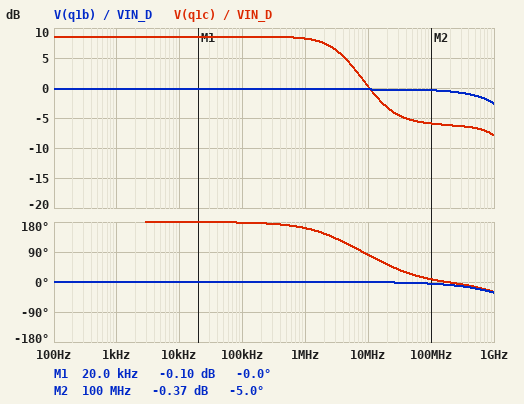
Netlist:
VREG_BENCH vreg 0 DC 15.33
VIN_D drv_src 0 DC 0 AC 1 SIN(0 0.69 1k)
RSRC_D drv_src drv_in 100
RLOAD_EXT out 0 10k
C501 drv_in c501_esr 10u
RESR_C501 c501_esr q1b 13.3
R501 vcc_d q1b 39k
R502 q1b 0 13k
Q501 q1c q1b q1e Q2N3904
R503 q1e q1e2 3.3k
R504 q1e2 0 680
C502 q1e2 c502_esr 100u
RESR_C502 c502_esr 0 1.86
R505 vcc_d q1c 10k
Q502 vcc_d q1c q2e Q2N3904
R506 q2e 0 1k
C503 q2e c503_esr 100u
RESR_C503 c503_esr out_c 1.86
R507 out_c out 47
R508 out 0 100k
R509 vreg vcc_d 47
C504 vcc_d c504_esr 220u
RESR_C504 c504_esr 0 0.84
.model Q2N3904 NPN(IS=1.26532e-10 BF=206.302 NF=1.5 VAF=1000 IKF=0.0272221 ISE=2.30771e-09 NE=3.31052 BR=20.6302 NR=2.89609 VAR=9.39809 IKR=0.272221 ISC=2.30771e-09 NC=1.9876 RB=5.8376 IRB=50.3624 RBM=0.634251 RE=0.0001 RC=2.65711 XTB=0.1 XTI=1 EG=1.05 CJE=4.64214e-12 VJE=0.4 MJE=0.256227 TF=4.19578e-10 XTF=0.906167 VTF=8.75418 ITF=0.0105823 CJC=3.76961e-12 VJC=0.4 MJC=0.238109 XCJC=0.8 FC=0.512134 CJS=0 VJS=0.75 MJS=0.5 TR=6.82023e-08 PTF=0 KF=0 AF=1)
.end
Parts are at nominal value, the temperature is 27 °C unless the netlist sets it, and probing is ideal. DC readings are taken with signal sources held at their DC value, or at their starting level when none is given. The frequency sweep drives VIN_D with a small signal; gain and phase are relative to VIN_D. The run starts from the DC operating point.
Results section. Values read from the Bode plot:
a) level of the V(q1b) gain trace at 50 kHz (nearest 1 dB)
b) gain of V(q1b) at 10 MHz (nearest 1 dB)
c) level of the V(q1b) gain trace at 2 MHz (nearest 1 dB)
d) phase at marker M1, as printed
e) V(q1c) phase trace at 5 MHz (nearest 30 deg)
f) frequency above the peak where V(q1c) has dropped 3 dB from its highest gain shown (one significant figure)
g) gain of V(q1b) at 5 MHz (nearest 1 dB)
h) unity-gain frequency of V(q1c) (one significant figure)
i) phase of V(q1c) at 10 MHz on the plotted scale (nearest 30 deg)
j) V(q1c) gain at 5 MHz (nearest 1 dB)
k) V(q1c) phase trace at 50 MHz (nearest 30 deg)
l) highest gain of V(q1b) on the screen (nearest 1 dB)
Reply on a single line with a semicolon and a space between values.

0 dB; 0 dB; 0 dB; -0.0 deg; 120 deg; 4 MHz; 0 dB; 10 MHz; 90 deg; 4 dB; 30 deg; 0 dB
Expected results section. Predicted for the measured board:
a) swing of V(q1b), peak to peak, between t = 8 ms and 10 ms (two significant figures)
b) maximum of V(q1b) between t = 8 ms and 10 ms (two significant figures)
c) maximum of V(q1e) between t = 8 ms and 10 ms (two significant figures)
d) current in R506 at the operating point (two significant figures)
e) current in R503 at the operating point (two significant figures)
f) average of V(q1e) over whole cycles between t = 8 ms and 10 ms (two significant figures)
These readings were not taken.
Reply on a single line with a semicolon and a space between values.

1.4 V; 4.4 V; 3.7 V; 6.2 mA; 770 µA; 3.1 V
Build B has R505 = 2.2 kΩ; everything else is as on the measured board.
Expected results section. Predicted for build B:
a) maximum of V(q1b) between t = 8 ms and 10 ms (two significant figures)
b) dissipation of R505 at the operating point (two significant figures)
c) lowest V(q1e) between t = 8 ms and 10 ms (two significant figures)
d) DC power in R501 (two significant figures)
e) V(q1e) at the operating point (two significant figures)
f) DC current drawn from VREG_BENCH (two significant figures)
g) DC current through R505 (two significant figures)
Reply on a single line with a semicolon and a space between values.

4.3 V; 1.6 mW; 2.3 V; 3.2 mW; 3.0 V; 13 mA; 850 µA
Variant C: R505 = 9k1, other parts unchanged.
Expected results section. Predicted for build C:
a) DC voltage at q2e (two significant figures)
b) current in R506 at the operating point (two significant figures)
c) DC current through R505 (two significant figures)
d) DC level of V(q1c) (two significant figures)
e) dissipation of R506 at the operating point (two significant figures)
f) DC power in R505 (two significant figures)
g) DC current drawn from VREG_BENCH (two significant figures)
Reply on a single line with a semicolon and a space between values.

6.8 V; 6.8 mA; 820 µA; 7.5 V; 47 mW; 6.1 mW; 7.9 mA
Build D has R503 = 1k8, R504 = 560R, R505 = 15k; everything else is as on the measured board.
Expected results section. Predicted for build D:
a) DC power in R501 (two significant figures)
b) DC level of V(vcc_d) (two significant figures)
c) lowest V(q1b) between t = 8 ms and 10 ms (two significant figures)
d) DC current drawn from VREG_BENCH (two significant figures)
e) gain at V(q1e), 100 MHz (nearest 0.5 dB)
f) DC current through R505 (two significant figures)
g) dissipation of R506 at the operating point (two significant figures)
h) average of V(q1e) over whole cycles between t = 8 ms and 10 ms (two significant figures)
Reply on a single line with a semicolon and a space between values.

3.9 mW; 15 V; 2.1 V; 2.8 mA; -1.0 dB; 860 µA; 2.8 mW; 2.2 V
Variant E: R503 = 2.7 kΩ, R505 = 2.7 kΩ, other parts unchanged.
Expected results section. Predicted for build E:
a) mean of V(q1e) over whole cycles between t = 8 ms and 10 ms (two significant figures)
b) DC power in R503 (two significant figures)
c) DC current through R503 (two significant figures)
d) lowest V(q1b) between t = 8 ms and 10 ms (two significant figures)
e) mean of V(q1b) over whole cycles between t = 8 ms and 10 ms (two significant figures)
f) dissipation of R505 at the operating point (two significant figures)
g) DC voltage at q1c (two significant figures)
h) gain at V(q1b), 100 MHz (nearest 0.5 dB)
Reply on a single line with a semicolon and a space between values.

3.0 V; 2.1 mW; 890 µA; 2.9 V; 3.6 V; 2.6 mW; 12 V; -0.5 dB
